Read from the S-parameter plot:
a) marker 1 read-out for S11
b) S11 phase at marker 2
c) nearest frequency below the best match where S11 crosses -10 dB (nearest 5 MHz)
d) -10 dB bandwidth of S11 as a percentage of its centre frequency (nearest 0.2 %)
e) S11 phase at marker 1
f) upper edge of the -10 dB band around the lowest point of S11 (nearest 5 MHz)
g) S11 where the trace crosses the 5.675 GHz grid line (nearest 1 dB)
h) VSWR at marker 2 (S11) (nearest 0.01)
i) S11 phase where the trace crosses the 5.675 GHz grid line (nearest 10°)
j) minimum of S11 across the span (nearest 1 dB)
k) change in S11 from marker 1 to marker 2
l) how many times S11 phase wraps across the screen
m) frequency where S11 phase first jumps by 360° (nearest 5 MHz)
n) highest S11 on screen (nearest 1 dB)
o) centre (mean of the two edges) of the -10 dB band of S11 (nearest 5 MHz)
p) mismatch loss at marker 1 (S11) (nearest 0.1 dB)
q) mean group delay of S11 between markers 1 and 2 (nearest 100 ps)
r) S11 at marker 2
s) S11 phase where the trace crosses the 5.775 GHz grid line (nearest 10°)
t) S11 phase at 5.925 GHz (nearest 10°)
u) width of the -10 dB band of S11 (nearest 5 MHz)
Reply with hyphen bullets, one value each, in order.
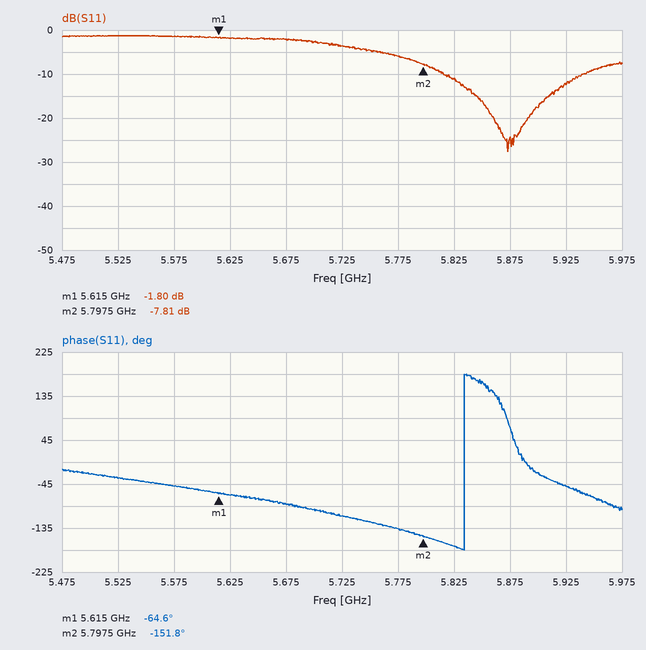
- -1.80 dB
- -151.8°
- 5.815 GHz
- 2.2 %
- -64.6°
- 5.940 GHz
- -2 dB
- 2.37
- -90°
- -28 dB
- -6.01 dB
- 1
- 5.835 GHz
- -1 dB
- 5.880 GHz
- 4.7 dB
- 1.3 ns
- -7.81 dB
- -140°
- -50°
- 125 MHz
